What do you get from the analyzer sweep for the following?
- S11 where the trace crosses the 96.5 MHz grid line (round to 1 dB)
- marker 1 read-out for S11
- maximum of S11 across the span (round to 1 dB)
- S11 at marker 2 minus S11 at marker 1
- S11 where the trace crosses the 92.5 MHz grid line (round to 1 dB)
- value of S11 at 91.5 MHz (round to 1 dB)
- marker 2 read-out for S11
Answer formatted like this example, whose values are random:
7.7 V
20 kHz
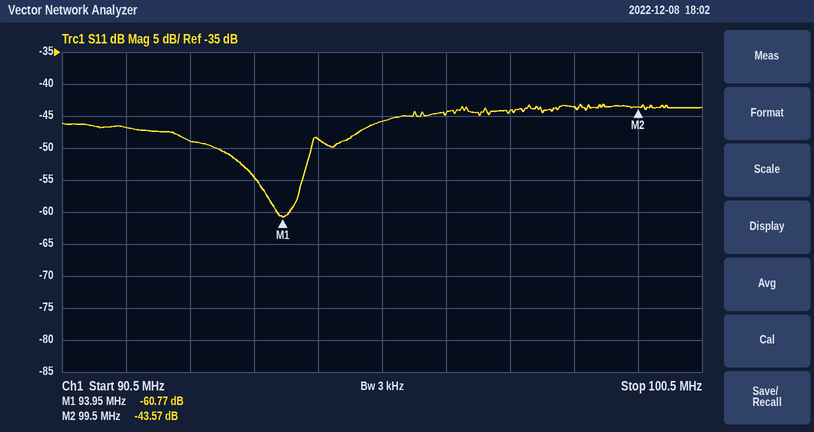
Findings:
-45 dB
-60.77 dB
-43 dB
17.20 dB
-49 dB
-47 dB
-43.57 dB
